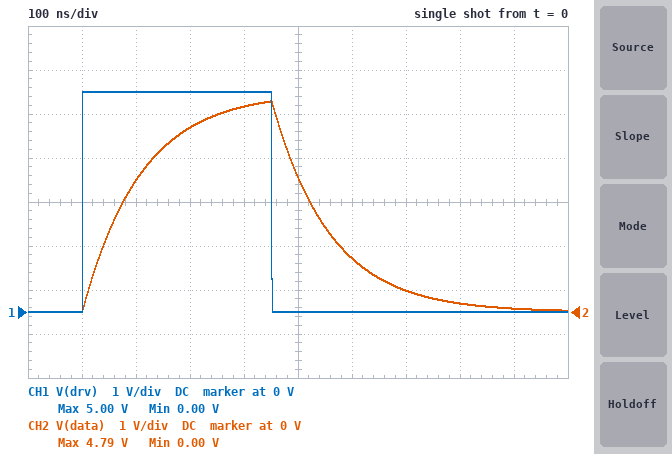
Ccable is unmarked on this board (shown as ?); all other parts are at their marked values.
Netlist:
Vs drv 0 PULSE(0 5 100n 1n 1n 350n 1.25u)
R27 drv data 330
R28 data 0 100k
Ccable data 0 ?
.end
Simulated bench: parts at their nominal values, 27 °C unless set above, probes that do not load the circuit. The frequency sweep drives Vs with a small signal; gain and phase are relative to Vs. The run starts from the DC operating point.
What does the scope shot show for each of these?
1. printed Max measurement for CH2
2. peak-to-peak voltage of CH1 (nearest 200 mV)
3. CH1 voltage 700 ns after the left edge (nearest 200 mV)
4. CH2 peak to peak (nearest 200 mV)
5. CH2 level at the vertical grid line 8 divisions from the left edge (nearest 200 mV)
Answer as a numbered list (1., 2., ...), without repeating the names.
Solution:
1. 4.79 V
2. 5.0 V
3. 0 V
4. 4.8 V
5. 200 mV
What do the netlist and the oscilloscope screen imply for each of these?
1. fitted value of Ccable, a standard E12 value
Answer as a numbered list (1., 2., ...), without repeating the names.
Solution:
1. 330 pF
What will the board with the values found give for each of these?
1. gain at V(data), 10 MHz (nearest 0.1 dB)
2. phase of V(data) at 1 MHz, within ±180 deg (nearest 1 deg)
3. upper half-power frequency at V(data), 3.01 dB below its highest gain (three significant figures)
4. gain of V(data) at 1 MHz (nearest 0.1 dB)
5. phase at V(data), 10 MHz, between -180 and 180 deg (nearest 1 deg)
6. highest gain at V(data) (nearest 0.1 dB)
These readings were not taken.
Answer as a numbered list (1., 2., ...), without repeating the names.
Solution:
1. -16.8 dB
2. -34 deg
3. 1.47 MHz
4. -1.7 dB
5. -82 deg
6. 0 dB
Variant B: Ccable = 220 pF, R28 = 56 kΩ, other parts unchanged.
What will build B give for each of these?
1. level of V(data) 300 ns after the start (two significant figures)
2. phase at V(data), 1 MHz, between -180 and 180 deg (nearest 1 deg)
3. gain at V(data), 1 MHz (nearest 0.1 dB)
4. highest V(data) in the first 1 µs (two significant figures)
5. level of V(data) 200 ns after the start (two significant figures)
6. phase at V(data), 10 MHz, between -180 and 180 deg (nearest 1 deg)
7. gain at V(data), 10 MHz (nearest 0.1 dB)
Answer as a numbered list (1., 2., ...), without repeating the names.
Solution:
1. 4.7 V
2. -24 deg
3. -0.9 dB
4. 4.9 V
5. 3.7 V
6. -78 deg
7. -13.4 dB
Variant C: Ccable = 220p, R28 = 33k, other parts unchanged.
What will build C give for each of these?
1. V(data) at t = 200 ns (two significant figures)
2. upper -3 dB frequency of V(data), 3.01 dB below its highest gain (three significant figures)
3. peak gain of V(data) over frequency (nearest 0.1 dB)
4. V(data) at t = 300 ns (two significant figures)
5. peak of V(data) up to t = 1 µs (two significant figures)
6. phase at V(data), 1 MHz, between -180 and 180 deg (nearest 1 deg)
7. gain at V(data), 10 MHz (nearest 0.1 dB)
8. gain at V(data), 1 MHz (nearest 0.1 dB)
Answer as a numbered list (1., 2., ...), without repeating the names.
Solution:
1. 3.7 V
2. 2.21 MHz
3. -0.1 dB
4. 4.6 V
5. 4.9 V
6. -24 deg
7. -13.4 dB
8. -0.9 dB
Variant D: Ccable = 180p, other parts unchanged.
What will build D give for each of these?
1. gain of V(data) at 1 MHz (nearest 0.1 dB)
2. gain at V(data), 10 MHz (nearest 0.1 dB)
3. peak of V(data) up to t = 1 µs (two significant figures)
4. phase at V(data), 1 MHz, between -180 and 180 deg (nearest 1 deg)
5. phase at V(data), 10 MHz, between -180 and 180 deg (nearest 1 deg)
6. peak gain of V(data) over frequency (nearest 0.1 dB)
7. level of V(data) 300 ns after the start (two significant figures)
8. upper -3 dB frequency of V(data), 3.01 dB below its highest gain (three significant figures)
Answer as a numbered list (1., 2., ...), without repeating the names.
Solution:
1. -0.6 dB
2. -11.7 dB
3. 5.0 V
4. -20 deg
5. -75 deg
6. 0 dB
7. 4.8 V
8. 2.69 MHz
